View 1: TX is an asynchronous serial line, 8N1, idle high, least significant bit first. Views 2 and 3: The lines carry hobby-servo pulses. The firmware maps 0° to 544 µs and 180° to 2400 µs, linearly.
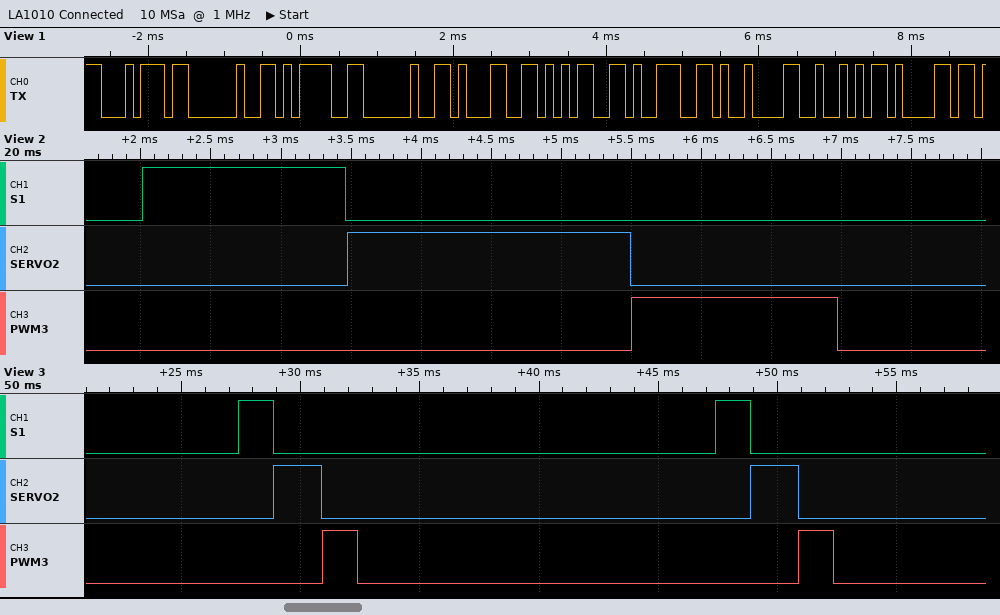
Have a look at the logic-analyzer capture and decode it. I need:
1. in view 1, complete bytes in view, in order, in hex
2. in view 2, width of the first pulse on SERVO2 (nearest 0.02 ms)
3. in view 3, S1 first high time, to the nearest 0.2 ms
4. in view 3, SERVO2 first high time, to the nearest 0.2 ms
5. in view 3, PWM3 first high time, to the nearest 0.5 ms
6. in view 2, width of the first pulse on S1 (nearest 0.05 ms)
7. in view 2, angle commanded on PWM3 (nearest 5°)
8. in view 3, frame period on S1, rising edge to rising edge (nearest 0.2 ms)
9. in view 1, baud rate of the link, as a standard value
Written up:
74 20 3D 20 31 35 39 09 52 61
2.02 ms
1.4 ms
2.0 ms
1.5 ms
1.45 ms
90°
20.0 ms
9600 baud
